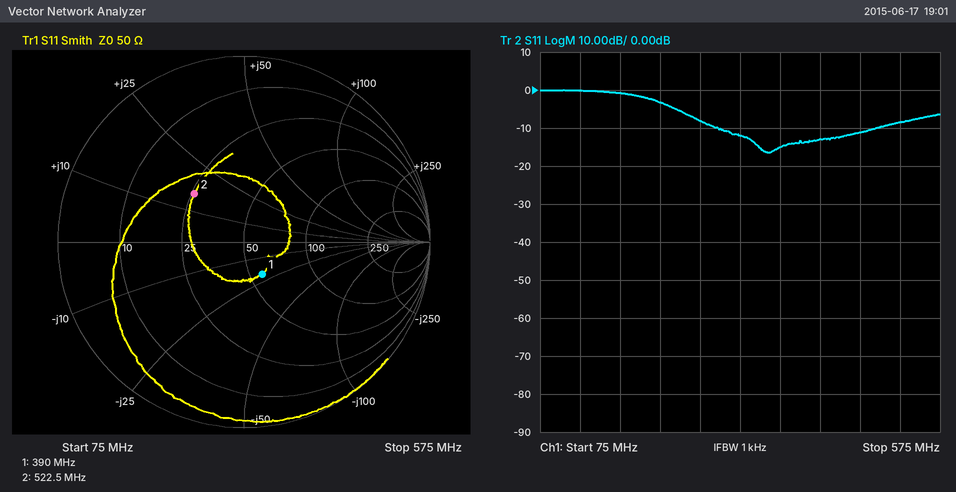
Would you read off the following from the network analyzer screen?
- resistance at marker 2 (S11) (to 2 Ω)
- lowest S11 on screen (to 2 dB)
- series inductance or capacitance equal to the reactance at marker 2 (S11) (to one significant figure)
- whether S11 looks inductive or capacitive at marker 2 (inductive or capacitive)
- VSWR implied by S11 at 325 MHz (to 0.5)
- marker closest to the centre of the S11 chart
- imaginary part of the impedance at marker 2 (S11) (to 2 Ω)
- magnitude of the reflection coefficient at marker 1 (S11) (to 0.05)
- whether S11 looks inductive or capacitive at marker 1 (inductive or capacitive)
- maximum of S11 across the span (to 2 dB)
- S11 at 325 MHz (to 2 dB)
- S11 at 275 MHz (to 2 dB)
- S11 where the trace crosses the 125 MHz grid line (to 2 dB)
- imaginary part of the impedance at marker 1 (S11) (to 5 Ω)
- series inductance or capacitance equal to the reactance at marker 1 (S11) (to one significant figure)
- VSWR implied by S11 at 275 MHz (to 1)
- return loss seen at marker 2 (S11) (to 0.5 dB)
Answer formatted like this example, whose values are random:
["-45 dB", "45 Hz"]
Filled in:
["26 Ω", "-16 dB", "5 nH", "inductive", "1.5", "marker 1", "+16 Ω", "0.20", "capacitive", "0 dB", "-12 dB", "-8 dB", "0 dB", "-20 Ω", "20 pF", "2", "8.5 dB"]
